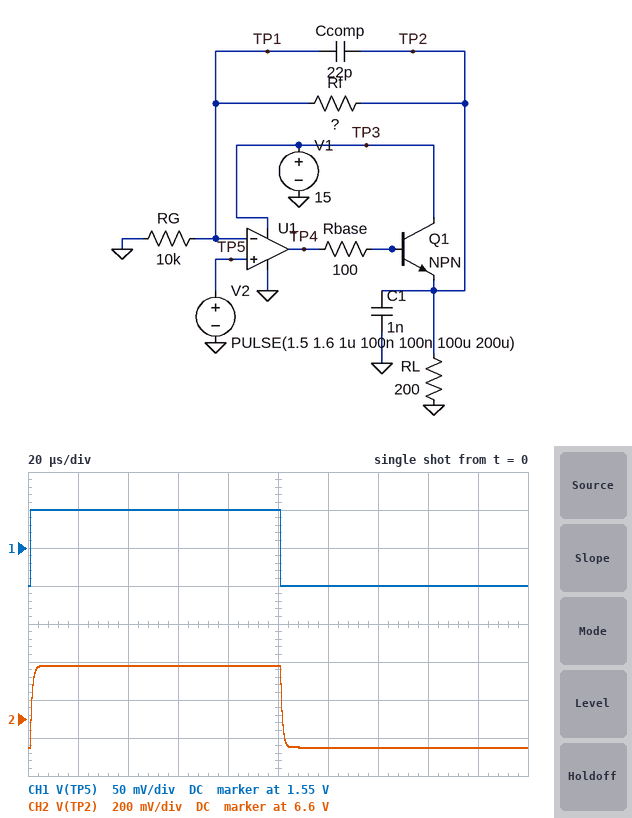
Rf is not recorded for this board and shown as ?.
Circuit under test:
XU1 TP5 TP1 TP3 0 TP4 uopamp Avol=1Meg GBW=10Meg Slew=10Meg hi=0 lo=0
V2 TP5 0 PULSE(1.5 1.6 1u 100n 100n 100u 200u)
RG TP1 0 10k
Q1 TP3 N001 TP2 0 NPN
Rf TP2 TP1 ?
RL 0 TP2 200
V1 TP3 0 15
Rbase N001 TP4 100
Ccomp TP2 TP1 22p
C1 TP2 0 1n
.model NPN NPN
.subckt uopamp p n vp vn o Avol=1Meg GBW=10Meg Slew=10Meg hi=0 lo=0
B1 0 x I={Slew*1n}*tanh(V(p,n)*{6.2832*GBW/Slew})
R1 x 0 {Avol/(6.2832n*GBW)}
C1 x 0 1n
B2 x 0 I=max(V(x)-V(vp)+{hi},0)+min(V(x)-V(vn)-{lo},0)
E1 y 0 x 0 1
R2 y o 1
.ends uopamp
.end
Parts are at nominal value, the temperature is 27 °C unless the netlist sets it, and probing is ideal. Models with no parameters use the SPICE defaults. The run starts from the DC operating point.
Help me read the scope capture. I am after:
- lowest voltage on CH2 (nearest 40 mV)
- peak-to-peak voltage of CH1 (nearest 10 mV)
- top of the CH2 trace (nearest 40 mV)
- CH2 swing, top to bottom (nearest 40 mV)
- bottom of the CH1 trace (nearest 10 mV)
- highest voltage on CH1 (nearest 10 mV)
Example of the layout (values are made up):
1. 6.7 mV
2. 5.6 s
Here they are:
1. 6.44 V
2. 100 mV
3. 6.88 V
4. 440 mV
5. 1.50 V
6. 1.60 V
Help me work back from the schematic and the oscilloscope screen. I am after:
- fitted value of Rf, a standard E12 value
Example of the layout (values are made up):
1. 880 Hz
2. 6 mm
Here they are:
1. 33 kΩ
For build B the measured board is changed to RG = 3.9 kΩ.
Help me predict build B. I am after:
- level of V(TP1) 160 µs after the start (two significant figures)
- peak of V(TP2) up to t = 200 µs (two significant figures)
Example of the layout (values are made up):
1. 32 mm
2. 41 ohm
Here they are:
1. 1.5 V
2. 14 V
